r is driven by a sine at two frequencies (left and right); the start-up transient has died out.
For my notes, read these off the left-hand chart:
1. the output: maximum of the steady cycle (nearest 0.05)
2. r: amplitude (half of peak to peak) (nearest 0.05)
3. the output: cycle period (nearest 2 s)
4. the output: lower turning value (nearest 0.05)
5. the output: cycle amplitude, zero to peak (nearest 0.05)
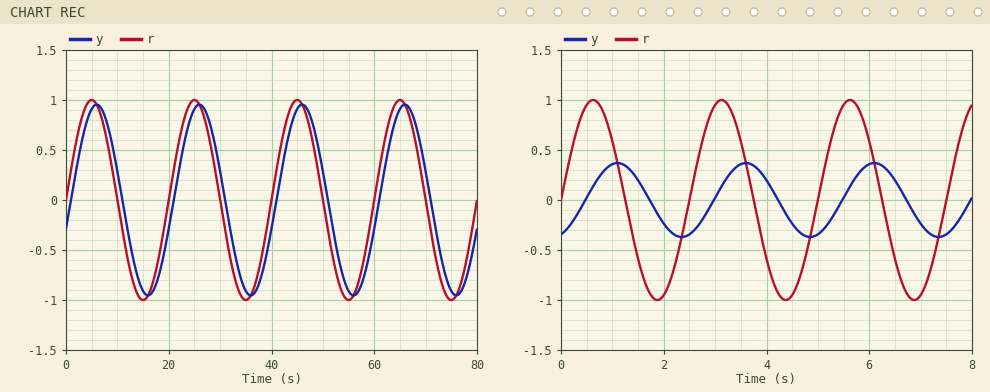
0.95
1.00
20 s
-0.95
0.95
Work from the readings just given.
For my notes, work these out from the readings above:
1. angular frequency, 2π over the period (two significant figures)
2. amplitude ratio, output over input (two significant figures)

0.31 rad/s
0.95
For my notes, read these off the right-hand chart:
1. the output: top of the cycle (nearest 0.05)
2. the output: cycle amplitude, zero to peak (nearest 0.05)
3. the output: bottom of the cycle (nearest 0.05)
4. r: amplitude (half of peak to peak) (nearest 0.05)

0.35
0.35
-0.35
1.00
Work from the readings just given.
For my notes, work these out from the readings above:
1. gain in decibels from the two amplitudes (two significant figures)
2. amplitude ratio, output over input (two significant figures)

-9.1 dB
0.35
